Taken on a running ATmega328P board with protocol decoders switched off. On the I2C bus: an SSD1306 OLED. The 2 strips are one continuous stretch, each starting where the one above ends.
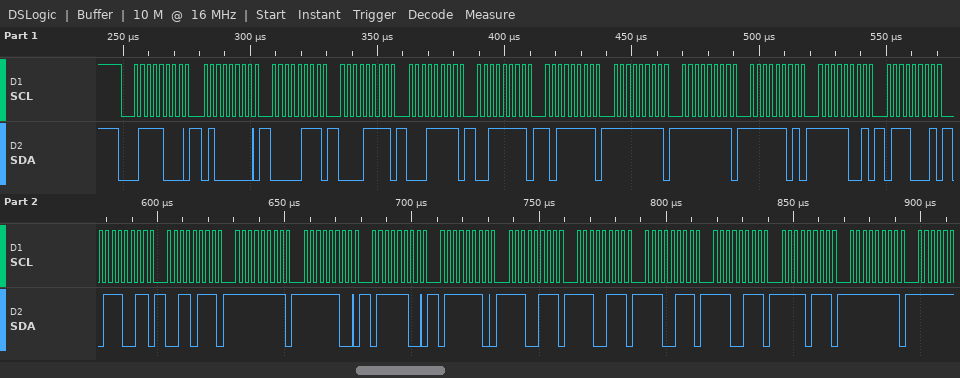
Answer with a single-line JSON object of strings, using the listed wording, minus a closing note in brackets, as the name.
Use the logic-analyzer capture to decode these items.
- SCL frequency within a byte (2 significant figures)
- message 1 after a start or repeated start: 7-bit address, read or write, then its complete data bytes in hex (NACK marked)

{"SCL frequency within a byte": "400 kHz", "message 1 after a start or repeated start: 7-bit address, read or write, then its complete data bytes in hex": "0x3C write: 40 07 0F 1F 3F BF FF FF FD F9 71 73 37 FF FC 7C 7E E7 E7 E7 E7 F7 FF"}
